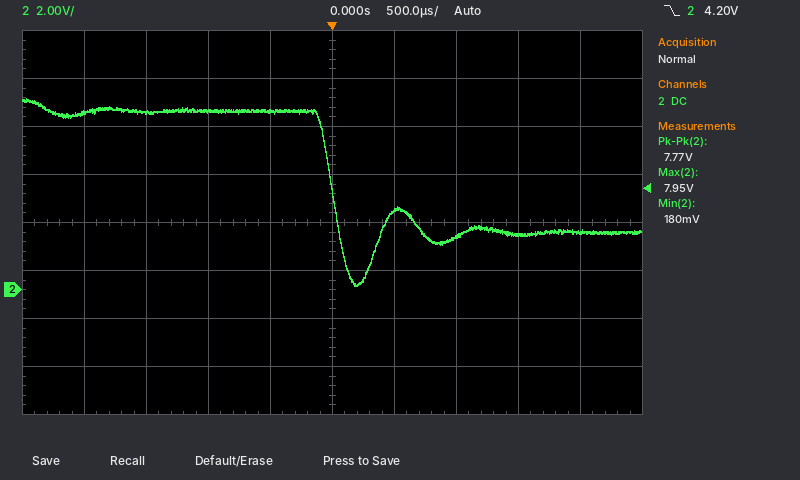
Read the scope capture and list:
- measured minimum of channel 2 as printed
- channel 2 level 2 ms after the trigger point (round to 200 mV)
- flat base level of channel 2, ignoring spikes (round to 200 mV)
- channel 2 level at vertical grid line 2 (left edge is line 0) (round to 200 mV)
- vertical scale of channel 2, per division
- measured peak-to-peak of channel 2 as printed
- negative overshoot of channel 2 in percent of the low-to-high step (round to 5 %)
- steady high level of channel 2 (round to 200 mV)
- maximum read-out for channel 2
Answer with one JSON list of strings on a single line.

["180 mV", "2.4 V", "2.4 V", "7.4 V", "2 V", "7.77 V", "45 %", "7.4 V", "7.95 V"]
